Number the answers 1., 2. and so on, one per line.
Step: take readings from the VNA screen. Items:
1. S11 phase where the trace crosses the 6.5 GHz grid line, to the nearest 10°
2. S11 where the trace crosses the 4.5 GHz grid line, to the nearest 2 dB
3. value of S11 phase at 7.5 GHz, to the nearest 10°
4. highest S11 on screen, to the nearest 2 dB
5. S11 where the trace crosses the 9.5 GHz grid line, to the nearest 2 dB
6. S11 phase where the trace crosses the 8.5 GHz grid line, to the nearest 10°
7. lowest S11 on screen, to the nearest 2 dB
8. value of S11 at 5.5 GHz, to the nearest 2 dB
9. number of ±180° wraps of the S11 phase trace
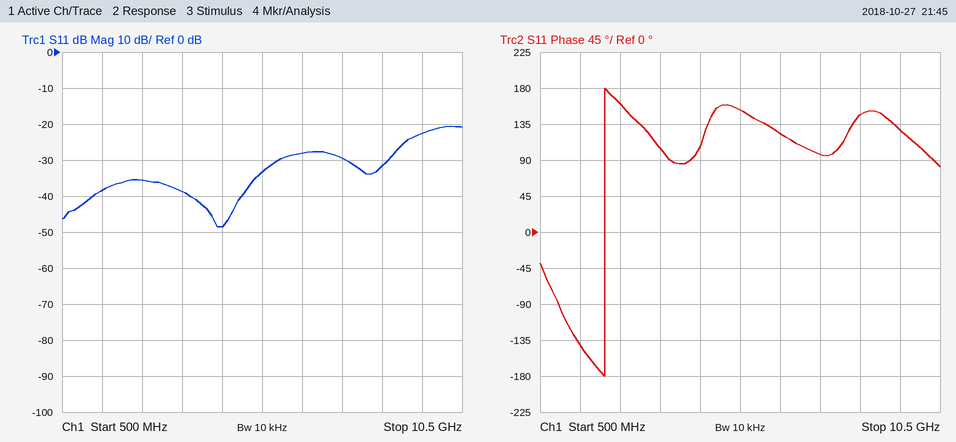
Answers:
1. 120°
2. -48 dB
3. 100°
4. -20 dB
5. -22 dB
6. 150°
7. -48 dB
8. -34 dB
9. 1
